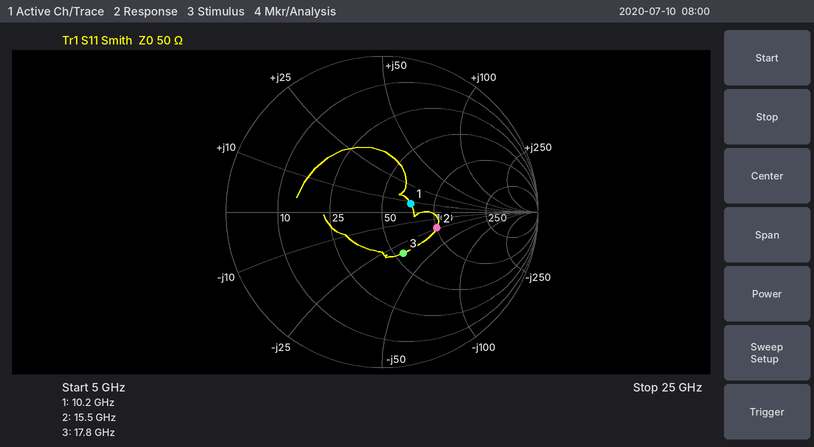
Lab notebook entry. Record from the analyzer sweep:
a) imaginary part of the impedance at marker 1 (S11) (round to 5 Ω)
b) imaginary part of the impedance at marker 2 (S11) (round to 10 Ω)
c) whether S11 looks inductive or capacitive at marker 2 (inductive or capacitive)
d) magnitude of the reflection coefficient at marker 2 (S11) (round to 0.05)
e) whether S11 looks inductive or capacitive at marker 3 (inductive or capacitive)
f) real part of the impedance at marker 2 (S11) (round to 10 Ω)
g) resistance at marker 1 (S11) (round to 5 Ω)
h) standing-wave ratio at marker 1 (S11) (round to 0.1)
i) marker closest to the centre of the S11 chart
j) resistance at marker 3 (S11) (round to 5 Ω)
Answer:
+10 Ω
-20 Ω
capacitive
0.35
capacitive
100 Ω
70 Ω
1.5
marker 1
55 Ω
